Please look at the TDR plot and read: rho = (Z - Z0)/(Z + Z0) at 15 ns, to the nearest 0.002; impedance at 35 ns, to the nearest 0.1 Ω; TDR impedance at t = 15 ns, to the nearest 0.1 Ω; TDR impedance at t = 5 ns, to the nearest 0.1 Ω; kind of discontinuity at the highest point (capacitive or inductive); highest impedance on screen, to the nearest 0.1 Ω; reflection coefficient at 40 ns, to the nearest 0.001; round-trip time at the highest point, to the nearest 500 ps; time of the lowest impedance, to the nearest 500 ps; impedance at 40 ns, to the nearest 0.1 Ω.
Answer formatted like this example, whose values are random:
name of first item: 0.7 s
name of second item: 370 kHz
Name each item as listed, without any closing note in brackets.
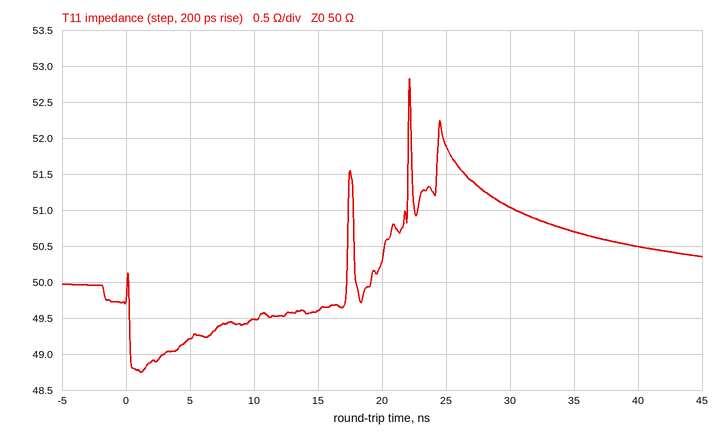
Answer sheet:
rho = (Z - Z0)/(Z + Z0) at 15 ns, to the nearest 0.002: -0.004
impedance at 35 ns, to the nearest 0.1 Ω: 50.7 Ω
TDR impedance at t = 15 ns, to the nearest 0.1 Ω: 49.6 Ω
TDR impedance at t = 5 ns, to the nearest 0.1 Ω: 49.2 Ω
kind of discontinuity at the highest point: inductive
highest impedance on screen, to the nearest 0.1 Ω: 52.8 Ω
reflection coefficient at 40 ns, to the nearest 0.001: +0.005
round-trip time at the highest point, to the nearest 500 ps: 22.0 ns
time of the lowest impedance, to the nearest 500 ps: 1.0 ns
impedance at 40 ns, to the nearest 0.1 Ω: 50.5 Ω
